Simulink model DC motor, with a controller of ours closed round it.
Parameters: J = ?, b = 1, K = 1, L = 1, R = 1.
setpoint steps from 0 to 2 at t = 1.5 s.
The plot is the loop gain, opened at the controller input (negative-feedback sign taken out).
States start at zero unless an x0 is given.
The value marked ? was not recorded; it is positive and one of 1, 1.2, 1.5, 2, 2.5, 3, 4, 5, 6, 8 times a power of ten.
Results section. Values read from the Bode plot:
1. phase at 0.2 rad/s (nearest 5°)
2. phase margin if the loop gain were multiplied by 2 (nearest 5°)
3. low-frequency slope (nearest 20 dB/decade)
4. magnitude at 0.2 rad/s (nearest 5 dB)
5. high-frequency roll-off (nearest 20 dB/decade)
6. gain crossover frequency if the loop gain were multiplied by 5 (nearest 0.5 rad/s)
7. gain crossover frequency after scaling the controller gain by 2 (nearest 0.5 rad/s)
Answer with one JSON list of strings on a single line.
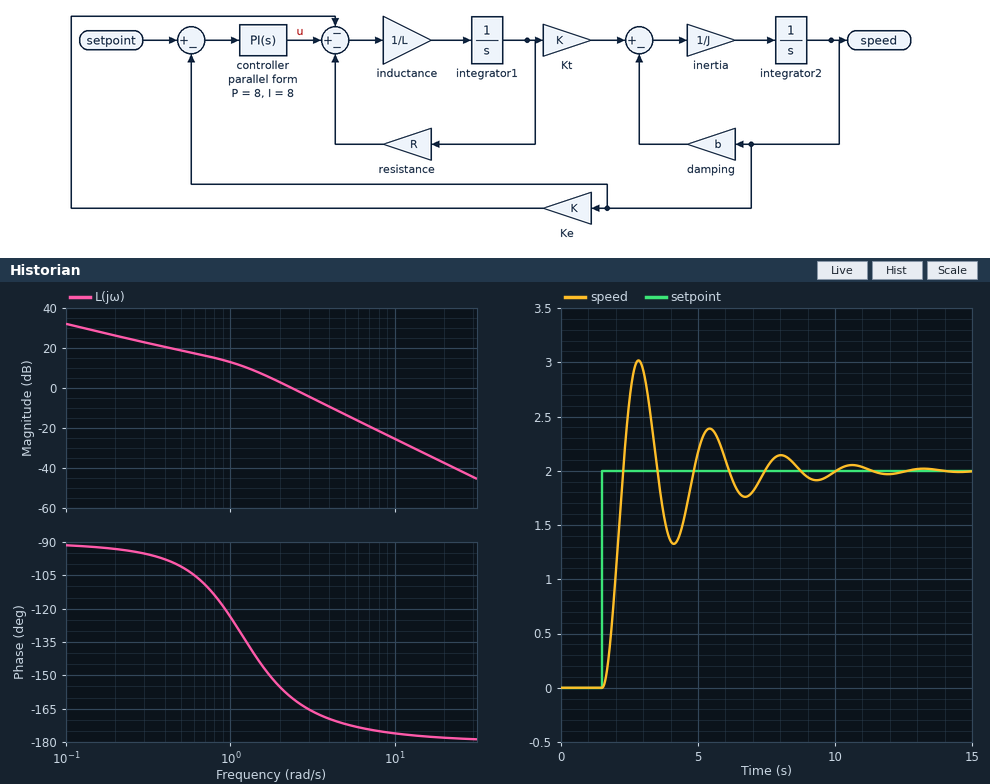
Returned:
["-95°", "15°", "-20 dB/decade", "25 dB", "-40 dB/decade", "5.0 rad/s", "3.5 rad/s"]
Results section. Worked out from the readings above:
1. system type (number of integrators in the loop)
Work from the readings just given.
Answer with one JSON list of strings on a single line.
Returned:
["1"]
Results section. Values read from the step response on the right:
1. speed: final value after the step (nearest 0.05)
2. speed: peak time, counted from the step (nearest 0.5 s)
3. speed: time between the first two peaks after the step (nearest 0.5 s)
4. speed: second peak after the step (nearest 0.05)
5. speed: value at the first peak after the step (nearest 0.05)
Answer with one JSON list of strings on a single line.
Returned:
["2.00", "1.5 s", "2.5 s", "2.40", "3.00"]
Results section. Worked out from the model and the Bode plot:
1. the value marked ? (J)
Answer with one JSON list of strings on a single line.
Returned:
["1.5"]
